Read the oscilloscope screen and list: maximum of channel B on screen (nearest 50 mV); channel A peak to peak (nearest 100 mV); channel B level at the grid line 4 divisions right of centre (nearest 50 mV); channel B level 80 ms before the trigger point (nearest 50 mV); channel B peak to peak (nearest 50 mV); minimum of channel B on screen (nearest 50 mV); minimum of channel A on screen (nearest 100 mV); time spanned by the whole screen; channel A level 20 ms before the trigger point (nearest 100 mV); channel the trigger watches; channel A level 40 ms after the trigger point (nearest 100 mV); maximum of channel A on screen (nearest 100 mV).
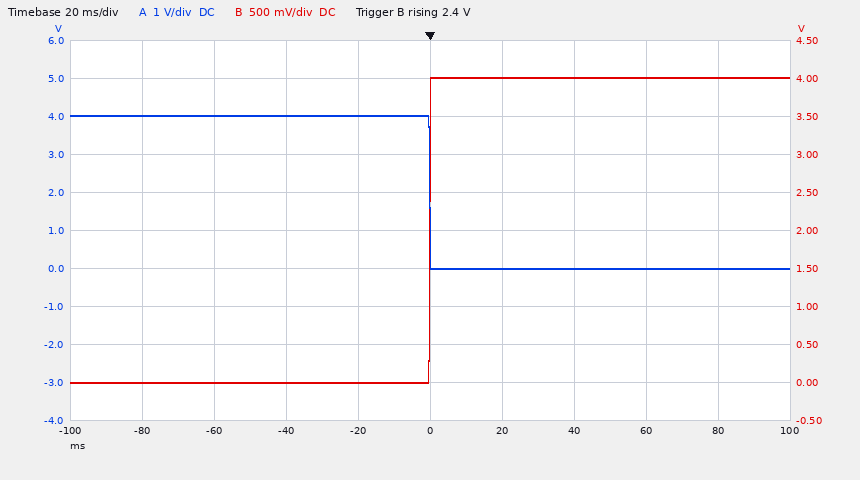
4.00 V
4.0 V
4.00 V
0 mV
4.00 V
0 mV
0.0 V
200 ms
4.0 V
channel B
0.0 V
4.0 V
